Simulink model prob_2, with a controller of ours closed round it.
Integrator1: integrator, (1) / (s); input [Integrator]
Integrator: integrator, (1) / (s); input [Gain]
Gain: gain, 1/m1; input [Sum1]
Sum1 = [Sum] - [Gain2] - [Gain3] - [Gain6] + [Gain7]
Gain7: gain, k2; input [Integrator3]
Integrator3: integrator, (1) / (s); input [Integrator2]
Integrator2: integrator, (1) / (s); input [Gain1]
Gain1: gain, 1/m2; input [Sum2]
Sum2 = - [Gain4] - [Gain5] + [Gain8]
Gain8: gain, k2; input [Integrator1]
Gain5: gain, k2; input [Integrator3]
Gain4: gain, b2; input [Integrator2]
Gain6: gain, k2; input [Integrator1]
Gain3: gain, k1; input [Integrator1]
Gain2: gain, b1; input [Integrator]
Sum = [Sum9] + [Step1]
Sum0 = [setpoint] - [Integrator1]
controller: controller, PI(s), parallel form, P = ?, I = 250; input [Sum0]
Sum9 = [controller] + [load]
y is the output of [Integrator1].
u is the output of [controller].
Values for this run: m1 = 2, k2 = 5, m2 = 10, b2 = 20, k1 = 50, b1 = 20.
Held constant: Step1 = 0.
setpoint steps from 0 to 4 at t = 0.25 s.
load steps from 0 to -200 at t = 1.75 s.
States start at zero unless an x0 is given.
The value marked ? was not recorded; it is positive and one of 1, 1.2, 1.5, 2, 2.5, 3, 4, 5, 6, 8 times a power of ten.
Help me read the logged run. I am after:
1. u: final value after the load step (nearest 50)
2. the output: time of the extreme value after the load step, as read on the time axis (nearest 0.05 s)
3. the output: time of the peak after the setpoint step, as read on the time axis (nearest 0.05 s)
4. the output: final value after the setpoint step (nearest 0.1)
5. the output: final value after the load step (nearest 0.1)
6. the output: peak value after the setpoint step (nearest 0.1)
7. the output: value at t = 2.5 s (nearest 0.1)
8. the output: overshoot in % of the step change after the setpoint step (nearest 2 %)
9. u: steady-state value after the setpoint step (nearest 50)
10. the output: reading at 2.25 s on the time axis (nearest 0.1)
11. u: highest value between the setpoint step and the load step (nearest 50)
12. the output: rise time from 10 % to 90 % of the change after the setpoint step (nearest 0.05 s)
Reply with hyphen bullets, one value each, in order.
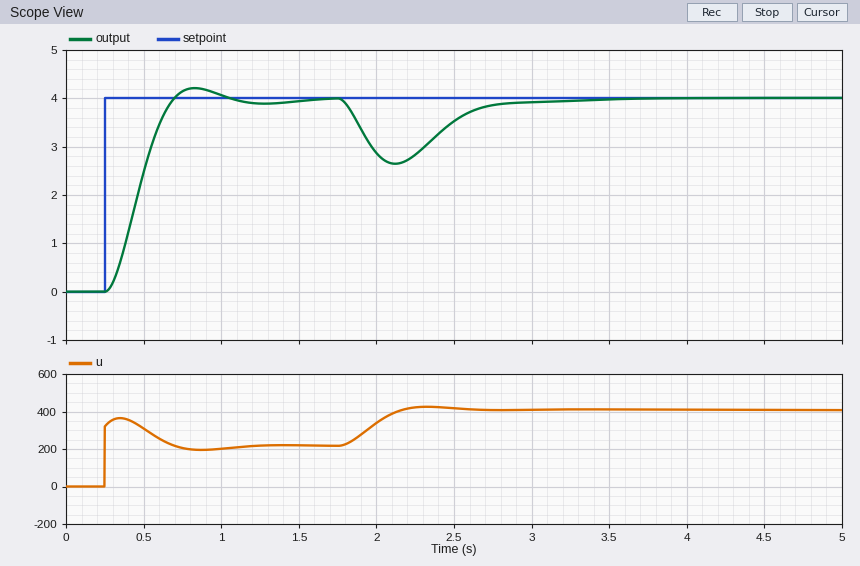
- 400
- 2.10 s
- 0.85 s
- 4.0
- 4.0
- 4.2
- 3.5
- 6 %
- 200
- 2.8
- 350
- 0.30 s
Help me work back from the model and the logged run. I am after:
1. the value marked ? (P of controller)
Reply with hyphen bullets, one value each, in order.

- 80
